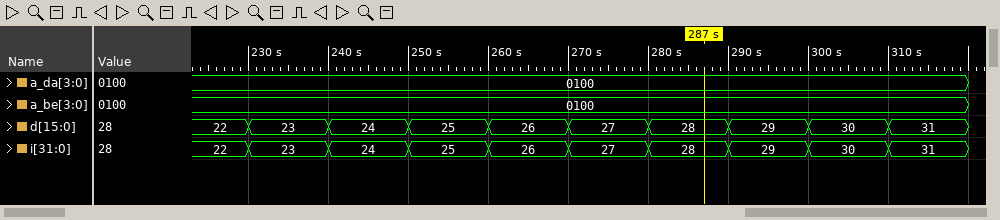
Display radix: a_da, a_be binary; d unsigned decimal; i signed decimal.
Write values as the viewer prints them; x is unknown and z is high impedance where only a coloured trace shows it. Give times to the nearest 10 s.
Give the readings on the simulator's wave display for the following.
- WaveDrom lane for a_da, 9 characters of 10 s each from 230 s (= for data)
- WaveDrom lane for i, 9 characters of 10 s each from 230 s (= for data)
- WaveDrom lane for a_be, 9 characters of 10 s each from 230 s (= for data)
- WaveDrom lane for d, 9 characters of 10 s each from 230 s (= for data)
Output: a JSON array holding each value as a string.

["{name: 'a_da', wave: '=........', data: '0100'}", "{name: 'i', wave: '=========', data: '23 24 25 26 27 28 29 30 31'}", "{name: 'a_be', wave: '=........', data: '0100'}", "{name: 'd', wave: '=========', data: '23 24 25 26 27 28 29 30 31'}"]
